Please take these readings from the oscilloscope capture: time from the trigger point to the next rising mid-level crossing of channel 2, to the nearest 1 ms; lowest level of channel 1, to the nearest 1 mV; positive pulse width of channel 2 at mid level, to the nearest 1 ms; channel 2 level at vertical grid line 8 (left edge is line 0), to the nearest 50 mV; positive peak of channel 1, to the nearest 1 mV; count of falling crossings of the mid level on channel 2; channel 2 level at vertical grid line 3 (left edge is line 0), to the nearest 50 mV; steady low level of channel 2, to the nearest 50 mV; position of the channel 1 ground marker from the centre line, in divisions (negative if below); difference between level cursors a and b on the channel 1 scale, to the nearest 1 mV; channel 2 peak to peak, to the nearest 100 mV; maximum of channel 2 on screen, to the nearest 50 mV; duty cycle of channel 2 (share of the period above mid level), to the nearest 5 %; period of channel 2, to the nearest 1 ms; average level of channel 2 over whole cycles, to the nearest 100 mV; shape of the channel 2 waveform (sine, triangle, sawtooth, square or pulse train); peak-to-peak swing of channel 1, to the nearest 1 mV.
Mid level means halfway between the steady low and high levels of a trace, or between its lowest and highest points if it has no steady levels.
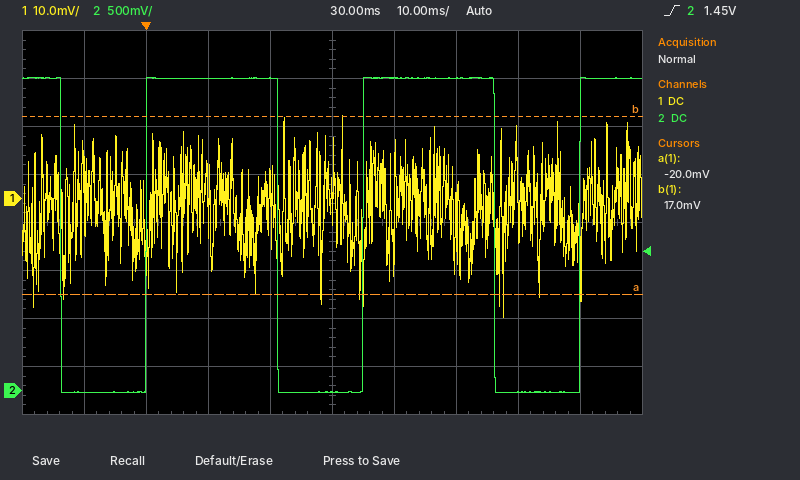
35 ms
-25 mV
21 ms
0 mV
17 mV
3
3.25 V
0 mV
+0.5 div
37 mV
3.30 V
3.25 V
60 %
35 ms
2.0 V
pulse train
42 mV
